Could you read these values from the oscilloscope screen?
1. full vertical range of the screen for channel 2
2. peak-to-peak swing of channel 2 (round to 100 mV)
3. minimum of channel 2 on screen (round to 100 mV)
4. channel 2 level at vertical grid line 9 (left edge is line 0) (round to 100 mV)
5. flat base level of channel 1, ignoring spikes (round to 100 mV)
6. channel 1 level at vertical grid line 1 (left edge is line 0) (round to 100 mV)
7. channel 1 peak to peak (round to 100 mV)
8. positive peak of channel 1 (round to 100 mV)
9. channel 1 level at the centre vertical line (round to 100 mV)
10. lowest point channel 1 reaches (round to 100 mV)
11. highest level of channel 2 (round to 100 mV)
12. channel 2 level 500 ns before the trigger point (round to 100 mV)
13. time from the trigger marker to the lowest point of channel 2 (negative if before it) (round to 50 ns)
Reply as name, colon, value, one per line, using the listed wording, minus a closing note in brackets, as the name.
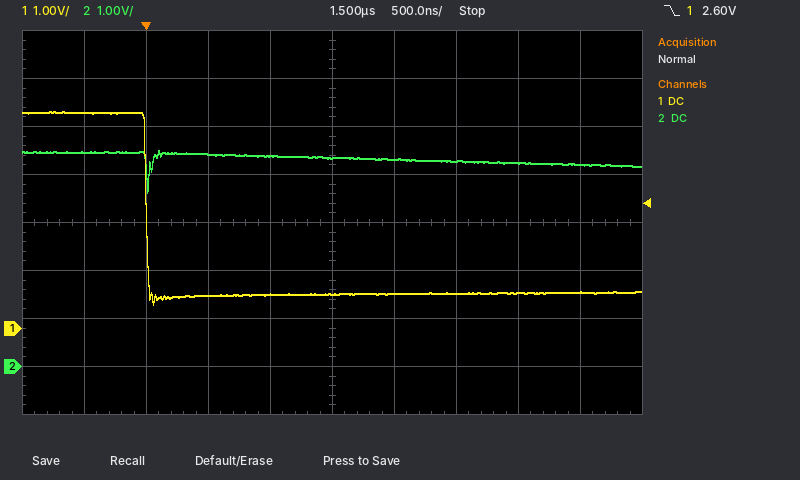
full vertical range of the screen for channel 2: 8 V
peak-to-peak swing of channel 2: 900 mV
minimum of channel 2 on screen: 3.6 V
channel 2 level at vertical grid line 9 (left edge is line 0): 4.2 V
flat base level of channel 1, ignoring spikes: 700 mV
channel 1 level at vertical grid line 1 (left edge is line 0): 4.5 V
channel 1 peak to peak: 4.0 V
positive peak of channel 1: 4.5 V
channel 1 level at the centre vertical line: 700 mV
lowest point channel 1 reaches: 500 mV
highest level of channel 2: 4.5 V
channel 2 level 500 ns before the trigger point: 4.5 V
time from the trigger marker to the lowest point of channel 2 (negative if before it): 0 ns
